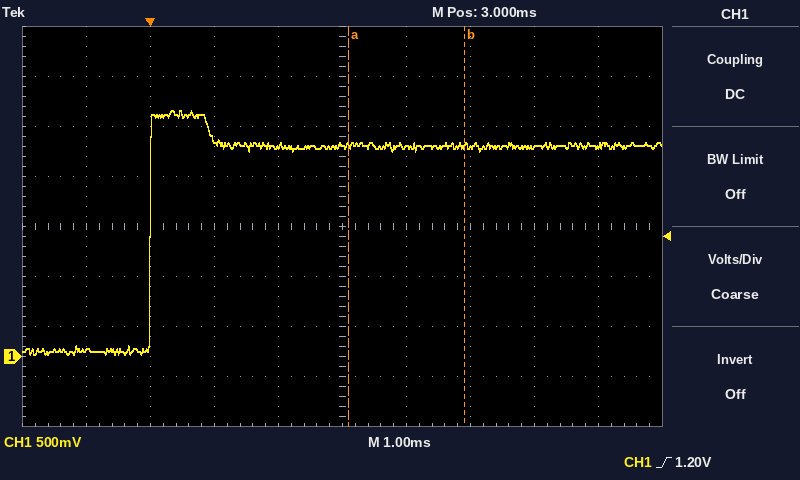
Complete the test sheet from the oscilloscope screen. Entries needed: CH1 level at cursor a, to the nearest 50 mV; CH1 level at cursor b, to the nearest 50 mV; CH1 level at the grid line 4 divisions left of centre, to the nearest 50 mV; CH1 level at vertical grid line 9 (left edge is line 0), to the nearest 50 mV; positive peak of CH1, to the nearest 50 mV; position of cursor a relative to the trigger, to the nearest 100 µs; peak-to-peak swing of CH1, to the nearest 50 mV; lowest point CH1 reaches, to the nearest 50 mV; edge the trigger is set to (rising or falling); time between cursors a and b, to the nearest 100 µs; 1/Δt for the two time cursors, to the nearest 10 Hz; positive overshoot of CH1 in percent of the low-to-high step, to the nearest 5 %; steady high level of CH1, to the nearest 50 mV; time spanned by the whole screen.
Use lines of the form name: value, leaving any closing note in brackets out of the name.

CH1 level at cursor a, to the nearest 50 mV: 2.10 V
CH1 level at cursor b, to the nearest 50 mV: 2.10 V
CH1 level at the grid line 4 divisions left of centre, to the nearest 50 mV: 50 mV
CH1 level at vertical grid line 9 (left edge is line 0), to the nearest 50 mV: 2.10 V
positive peak of CH1, to the nearest 50 mV: 2.45 V
position of cursor a relative to the trigger, to the nearest 100 µs: +3.1 ms
peak-to-peak swing of CH1, to the nearest 50 mV: 2.45 V
lowest point CH1 reaches, to the nearest 50 mV: 0 mV
edge the trigger is set to: rising
time between cursors a and b, to the nearest 100 µs: 1.8 ms
1/Δt for the two time cursors, to the nearest 10 Hz: 560 Hz
positive overshoot of CH1 in percent of the low-to-high step, to the nearest 5 %: 15 %
steady high level of CH1, to the nearest 50 mV: 2.10 V
time spanned by the whole screen: 10 ms
